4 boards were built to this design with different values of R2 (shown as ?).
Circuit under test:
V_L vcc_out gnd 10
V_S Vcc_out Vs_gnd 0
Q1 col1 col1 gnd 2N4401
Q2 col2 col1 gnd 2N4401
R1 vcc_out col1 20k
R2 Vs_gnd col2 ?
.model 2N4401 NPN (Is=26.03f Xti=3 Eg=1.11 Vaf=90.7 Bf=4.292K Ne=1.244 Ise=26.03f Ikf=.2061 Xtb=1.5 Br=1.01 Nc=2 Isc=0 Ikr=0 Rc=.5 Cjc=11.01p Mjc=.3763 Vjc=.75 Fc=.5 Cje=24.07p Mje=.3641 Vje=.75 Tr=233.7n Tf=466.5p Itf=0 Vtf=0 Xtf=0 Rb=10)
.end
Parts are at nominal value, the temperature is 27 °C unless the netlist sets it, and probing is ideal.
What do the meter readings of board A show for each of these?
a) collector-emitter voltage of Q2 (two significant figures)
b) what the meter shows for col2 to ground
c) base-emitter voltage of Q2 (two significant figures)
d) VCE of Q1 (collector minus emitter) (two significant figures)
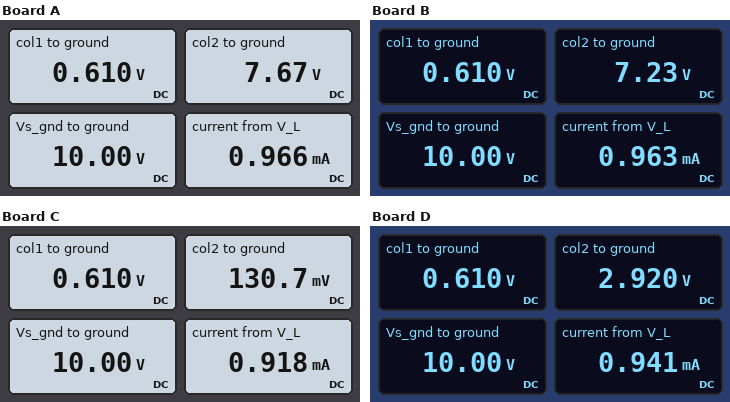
7.7 V
7.67 V
610 mV
610 mV
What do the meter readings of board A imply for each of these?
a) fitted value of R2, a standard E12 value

4.7 kΩ
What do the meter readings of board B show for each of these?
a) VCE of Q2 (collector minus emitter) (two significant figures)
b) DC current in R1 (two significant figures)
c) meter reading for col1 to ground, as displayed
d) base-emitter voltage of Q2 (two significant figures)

7.2 V
470 µA
0.610 V
610 mV
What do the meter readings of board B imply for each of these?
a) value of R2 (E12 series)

5.6 kΩ
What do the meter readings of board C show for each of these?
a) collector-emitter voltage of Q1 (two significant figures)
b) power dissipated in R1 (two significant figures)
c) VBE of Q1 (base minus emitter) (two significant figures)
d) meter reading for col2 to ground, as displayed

610 mV
4.4 mW
610 mV
130.7 mV
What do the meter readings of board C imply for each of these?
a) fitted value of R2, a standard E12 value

22 kΩ
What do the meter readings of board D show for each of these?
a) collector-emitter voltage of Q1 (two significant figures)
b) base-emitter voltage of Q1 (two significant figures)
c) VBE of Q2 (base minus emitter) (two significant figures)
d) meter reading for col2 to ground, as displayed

610 mV
610 mV
610 mV
2.920 V
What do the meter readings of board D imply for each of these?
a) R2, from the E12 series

15 kΩ
